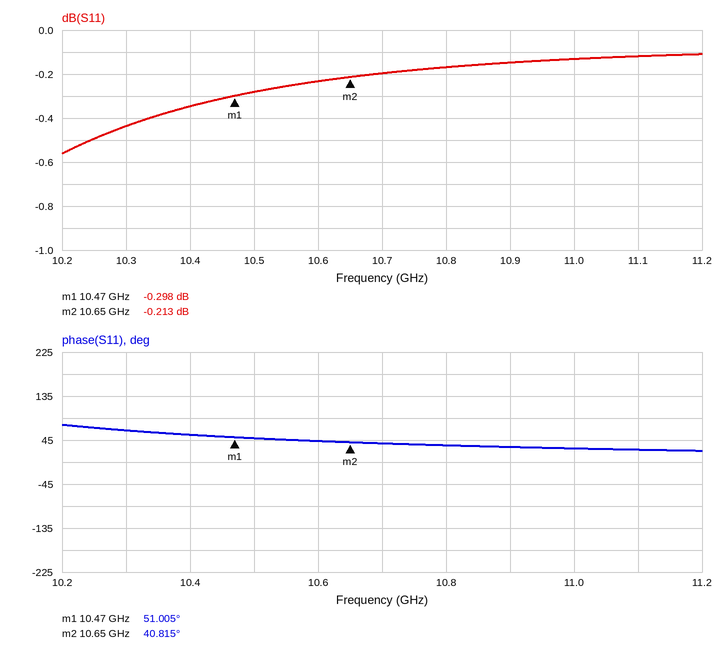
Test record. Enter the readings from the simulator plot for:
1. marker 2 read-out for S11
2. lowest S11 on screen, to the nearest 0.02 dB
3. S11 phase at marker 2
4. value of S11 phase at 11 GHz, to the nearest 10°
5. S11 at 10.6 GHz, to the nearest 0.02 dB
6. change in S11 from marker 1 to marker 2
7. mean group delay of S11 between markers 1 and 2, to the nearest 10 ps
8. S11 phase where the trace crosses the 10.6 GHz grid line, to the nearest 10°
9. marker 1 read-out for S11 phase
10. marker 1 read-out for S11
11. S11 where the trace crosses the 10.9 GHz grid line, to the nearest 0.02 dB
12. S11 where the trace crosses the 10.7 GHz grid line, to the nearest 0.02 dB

-0.213 dB
-0.56 dB
40.815°
30°
-0.24 dB
0.085 dB
160 ps
40°
51.005°
-0.298 dB
-0.14 dB
-0.20 dB
